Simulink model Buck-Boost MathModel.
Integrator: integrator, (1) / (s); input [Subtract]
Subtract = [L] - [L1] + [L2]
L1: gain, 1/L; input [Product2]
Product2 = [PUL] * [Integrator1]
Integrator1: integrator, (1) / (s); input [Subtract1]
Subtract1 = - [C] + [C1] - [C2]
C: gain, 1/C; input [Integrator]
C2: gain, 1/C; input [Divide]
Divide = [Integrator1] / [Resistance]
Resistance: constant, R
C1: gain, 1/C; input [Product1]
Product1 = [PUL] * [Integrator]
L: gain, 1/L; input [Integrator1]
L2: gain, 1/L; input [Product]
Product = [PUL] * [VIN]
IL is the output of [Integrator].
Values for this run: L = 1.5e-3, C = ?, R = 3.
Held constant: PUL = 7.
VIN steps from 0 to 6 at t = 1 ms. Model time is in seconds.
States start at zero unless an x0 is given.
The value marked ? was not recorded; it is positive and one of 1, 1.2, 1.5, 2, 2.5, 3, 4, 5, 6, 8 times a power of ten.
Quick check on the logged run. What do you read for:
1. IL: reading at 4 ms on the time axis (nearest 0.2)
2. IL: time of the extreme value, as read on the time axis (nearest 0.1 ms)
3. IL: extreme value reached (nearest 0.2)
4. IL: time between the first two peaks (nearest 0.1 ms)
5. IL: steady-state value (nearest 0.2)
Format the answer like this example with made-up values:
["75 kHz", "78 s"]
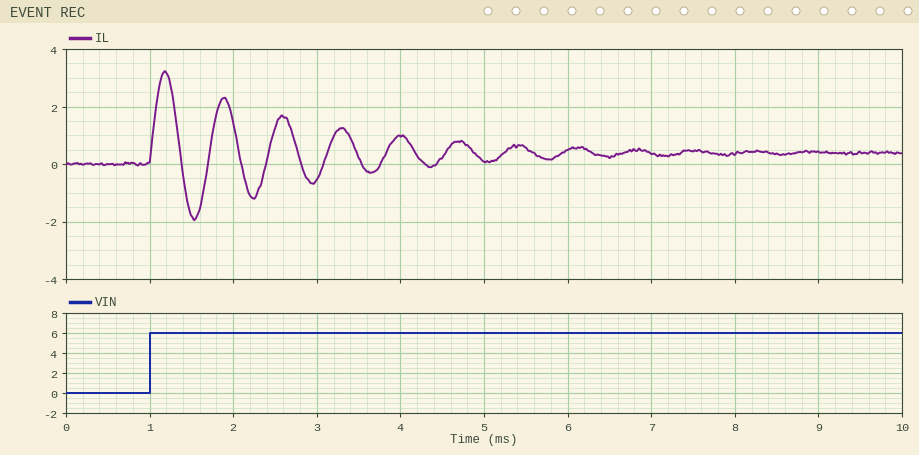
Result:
["1.0", "1.2 ms", "3.2", "0.7 ms", "0.4"]
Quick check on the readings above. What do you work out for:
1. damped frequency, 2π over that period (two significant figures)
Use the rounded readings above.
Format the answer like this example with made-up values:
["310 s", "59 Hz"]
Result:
["9.0 rad/ms"]
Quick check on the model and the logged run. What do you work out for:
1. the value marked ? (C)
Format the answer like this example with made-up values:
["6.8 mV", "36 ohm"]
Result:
["0.0003"]
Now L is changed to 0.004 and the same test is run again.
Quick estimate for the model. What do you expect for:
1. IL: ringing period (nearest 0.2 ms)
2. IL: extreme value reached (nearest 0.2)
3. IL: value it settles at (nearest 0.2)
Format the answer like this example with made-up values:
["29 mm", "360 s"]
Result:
["1.2 ms", "2.0", "0.4"]
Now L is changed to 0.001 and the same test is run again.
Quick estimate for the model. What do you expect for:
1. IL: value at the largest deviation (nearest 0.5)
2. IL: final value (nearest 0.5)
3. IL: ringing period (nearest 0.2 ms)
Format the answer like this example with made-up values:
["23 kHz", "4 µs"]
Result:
["4.0", "0.5", "0.6 ms"]
